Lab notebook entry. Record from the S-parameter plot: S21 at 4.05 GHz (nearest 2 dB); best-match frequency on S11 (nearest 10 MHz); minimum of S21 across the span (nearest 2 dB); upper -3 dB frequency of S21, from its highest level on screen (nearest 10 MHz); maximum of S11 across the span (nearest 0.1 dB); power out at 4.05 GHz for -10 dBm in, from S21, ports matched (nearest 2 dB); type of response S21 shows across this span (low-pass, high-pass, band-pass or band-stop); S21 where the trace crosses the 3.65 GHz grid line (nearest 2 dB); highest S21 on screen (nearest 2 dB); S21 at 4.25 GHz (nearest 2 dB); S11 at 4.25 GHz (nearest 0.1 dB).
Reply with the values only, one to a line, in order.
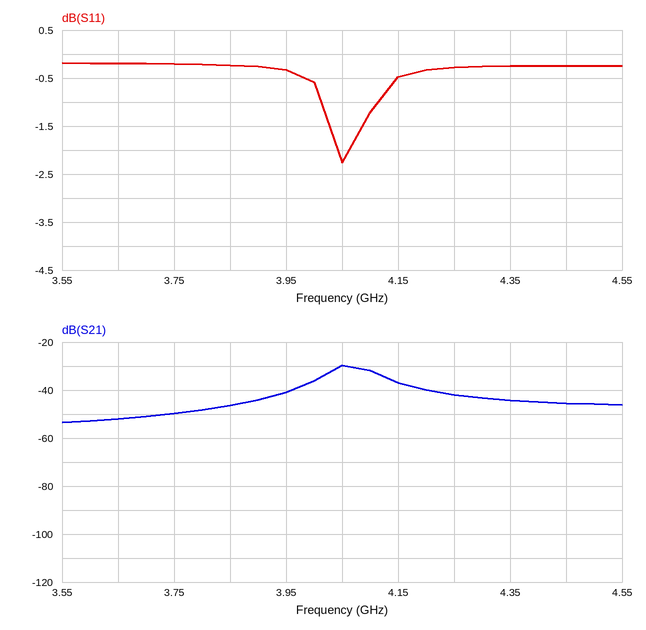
-30 dB
4.05 GHz
-54 dB
4.11 GHz
-0.2 dB
-40 dBm
band-pass
-52 dB
-30 dB
-42 dB
-0.3 dB
